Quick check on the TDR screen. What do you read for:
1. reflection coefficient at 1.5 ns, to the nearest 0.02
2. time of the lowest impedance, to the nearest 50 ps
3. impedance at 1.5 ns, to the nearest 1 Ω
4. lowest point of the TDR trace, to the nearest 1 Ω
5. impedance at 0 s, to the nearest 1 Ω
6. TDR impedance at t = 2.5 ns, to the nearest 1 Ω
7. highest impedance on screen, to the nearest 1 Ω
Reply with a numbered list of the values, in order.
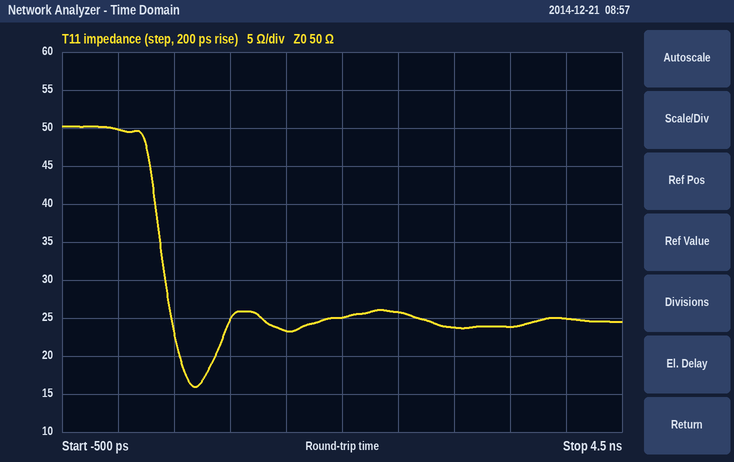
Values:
1. -0.36
2. 700 ps
3. 23 Ω
4. 16 Ω
5. 50 Ω
6. 26 Ω
7. 50 Ω
